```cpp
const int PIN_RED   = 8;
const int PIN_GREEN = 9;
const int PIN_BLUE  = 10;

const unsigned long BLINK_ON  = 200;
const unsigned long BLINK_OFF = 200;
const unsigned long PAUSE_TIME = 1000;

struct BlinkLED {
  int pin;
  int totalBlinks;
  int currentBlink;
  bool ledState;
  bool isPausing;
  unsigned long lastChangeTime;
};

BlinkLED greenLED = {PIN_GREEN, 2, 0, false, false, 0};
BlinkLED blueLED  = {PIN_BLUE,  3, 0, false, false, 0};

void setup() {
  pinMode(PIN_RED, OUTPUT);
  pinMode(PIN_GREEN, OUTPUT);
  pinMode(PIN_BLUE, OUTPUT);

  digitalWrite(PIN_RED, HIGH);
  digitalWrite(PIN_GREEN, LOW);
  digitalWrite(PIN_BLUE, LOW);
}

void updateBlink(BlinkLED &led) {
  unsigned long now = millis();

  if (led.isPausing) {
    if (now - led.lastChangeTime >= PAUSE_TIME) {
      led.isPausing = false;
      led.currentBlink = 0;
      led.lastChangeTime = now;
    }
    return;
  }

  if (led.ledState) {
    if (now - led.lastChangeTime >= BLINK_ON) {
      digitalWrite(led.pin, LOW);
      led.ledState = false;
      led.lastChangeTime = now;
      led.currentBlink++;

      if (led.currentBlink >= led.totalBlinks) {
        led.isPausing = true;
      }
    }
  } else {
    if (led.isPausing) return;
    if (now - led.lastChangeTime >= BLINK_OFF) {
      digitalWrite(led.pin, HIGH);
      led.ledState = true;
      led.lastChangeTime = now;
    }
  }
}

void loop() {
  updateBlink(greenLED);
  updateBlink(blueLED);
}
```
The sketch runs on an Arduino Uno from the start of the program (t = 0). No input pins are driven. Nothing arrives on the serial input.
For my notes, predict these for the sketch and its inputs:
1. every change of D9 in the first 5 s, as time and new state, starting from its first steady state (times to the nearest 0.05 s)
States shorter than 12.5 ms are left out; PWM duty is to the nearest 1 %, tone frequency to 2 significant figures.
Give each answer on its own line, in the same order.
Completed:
0 s low; 0.2 s high; 0.4 s low; 0.6 s high; 0.8 s low; 2 s high; 2.2 s low; 2.4 s high; 2.6 s low; 3.8 s high; 4 s low; 4.2 s high; 4.4 s low
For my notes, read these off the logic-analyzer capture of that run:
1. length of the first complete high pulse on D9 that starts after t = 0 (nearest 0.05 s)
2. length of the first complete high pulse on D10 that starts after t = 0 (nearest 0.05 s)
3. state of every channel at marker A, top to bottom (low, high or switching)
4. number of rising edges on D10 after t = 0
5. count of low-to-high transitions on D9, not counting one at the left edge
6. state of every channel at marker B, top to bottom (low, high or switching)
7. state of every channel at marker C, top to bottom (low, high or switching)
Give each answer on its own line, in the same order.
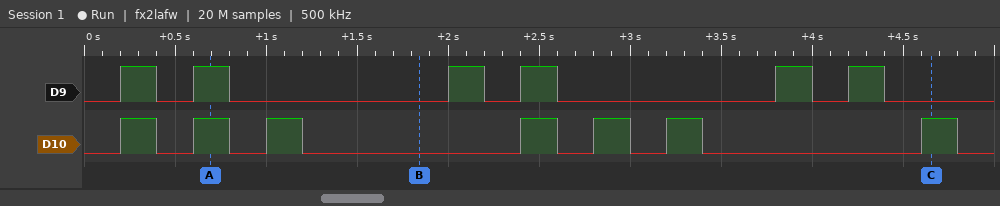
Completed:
0.20 s
0.20 s
D9 high, D10 high
7
6
D9 low, D10 low
D9 low, D10 high
